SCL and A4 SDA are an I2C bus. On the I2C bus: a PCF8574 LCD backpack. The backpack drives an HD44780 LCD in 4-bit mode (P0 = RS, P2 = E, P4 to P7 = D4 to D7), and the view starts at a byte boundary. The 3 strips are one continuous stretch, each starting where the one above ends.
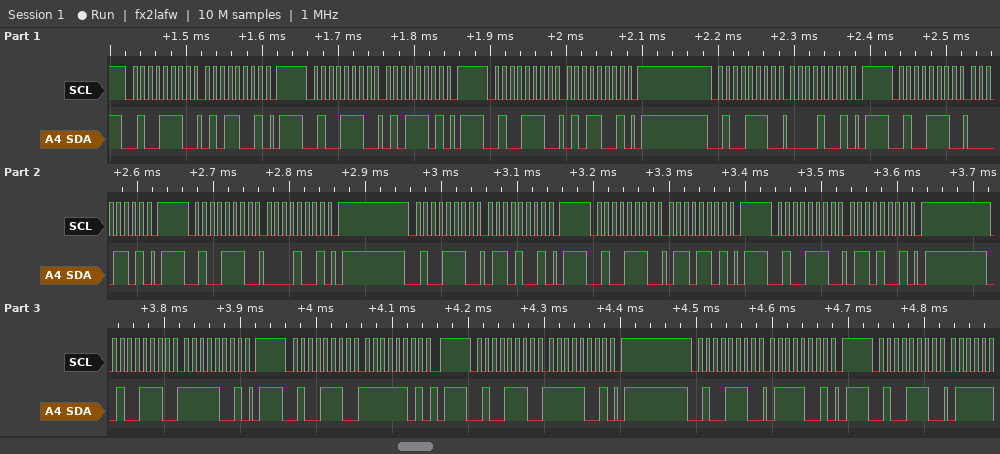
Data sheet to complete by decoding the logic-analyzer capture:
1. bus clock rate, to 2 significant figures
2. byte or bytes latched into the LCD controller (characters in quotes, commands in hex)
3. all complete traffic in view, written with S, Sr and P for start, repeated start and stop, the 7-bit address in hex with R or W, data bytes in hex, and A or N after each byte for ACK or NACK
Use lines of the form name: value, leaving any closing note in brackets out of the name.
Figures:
bus clock rate, to 2 significant figures: 100 kHz
byte or bytes latched into the LCD controller: 'P' 'o'
all complete traffic in view, written with S, Sr and P for start, repeated start and stop, the 7-bit address in hex with R or W, data bytes in hex, and A or N after each byte for ACK or NACK: S 27W A 59 A P S 27W A 5D A P S 27W A 59 A P S 27W A 09 A P S 27W A 0D A P S 27W A 09 A P S 27W A 69 A P S 27W A 6D A P S 27W A 69 A P S 27W A F9 A P S 27W A FD A P S 27W A F9 A P S 27W A 79 A P S 27W A
